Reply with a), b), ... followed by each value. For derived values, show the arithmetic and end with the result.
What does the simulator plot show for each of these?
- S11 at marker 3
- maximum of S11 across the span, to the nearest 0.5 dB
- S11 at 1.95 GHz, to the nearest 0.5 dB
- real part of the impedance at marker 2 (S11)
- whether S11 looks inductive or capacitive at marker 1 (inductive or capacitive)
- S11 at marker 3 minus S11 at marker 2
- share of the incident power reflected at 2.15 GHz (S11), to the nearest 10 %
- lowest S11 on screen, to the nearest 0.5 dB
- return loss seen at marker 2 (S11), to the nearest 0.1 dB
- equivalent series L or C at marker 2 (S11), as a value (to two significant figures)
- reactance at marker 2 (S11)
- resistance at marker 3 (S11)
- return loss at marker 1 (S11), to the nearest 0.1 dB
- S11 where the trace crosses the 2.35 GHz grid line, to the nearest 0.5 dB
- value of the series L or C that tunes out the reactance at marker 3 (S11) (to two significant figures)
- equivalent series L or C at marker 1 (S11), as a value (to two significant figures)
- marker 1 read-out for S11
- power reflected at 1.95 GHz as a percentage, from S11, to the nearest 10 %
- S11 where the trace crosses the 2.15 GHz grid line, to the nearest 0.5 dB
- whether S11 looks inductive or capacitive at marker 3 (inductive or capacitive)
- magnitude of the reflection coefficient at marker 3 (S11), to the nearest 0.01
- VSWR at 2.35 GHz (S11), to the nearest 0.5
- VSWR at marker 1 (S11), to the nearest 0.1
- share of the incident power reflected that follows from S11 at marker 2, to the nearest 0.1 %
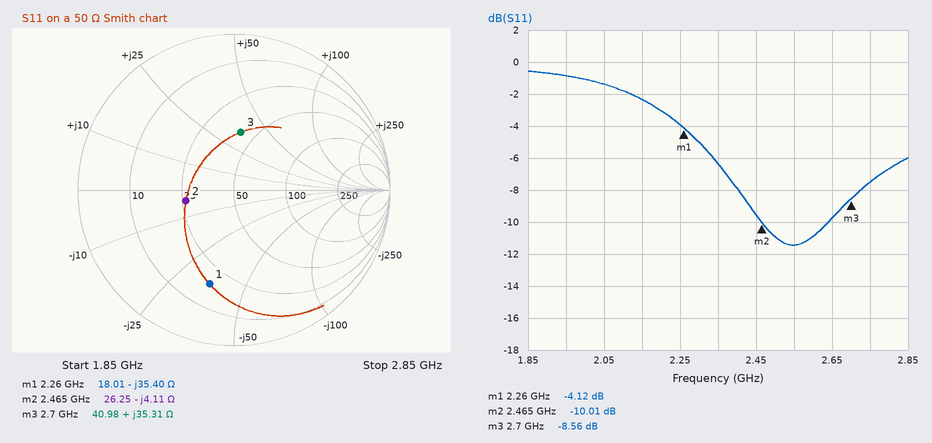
a) -8.56 dB
b) -0.5 dB
c) -1.0 dB
d) 26.25 Ω
e) capacitive
f) -8.56 − (-10.01) = 1.45 dB
g) 10^(-2.5/10) ≈ 56.2 %, so 60 % to the nearest 10 %
h) -11.5 dB
i) 10.0 dB
j) C = 1/(2π × 2.465 GHz × 4.11 Ω) ≈ 16 pF
k) -4.11 Ω
l) 40.98 Ω
m) 4.1 dB
n) -6.5 dB
o) C = 1/(2π × 2.7 GHz × 35.31 Ω) ≈ 1.7 pF
p) C = 1/(2π × 2.26 GHz × 35.4 Ω) ≈ 2.0 pF
q) -4.12 dB
r) 10^(-1/10) ≈ 79.4 %, so 80 % to the nearest 10 %
s) -2.5 dB
t) inductive
u) 10^(-8.56/20) ≈ 0.37
v) |Γ| = 10^(-6.5/20) = 0.4732; VSWR = (1 + 0.4732)/(1 − 0.4732) ≈ 2.80, so 3.0 to the nearest 0.5
w) (1 + 0.6223)/(1 − 0.6223) ≈ 4.3
x) 10^(-10.01/10) ≈ 10.0 %
